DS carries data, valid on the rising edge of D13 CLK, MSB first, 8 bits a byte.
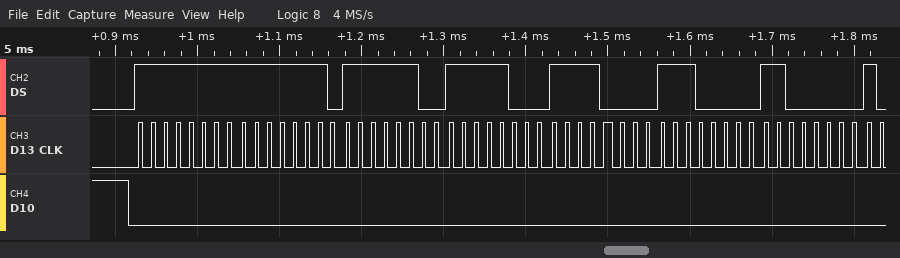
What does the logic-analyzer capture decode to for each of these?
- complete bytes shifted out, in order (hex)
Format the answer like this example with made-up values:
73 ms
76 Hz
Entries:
0xFF 0xFE 0xFC 0xF8 0xF0 0xE0 0xC0
